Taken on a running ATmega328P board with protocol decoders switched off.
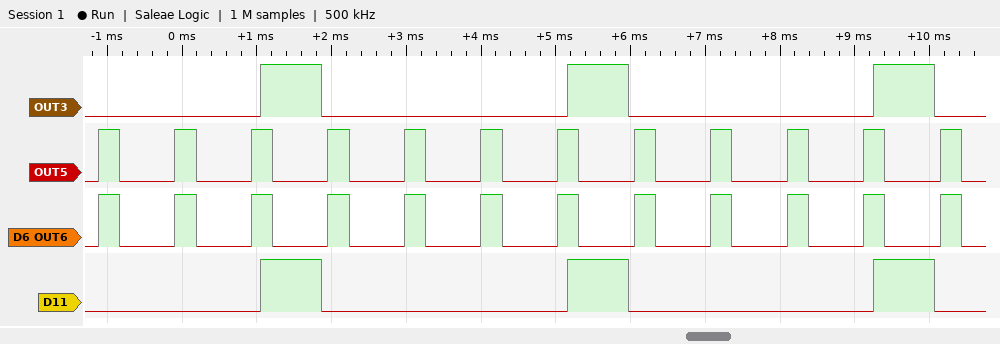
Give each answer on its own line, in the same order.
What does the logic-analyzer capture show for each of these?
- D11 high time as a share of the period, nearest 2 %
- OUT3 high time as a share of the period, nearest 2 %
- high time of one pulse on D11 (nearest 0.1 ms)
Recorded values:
20 %
20 %
0.8 ms
